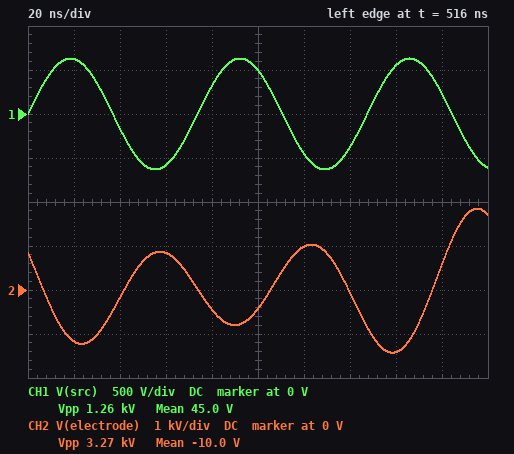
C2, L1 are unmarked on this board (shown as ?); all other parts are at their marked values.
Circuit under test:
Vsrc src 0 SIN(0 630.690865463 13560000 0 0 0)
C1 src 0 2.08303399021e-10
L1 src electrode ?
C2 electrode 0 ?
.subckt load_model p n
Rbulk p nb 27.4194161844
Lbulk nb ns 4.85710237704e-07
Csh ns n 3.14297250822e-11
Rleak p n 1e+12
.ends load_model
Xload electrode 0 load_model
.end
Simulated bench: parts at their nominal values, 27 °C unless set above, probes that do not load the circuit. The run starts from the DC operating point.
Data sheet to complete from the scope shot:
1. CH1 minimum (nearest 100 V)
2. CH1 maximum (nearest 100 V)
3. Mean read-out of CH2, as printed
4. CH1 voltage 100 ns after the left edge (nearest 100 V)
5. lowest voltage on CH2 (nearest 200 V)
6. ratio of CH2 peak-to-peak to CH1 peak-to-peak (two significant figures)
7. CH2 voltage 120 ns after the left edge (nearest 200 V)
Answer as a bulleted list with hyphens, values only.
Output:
- -600 V
- 600 V
- -10.0 V
- 500 V
- -1.4 kV
- 2.6
- 1.0 kV
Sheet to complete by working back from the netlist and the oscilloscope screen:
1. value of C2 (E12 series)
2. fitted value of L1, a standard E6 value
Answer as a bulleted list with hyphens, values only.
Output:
- 47 pF
- 2.2 µH
